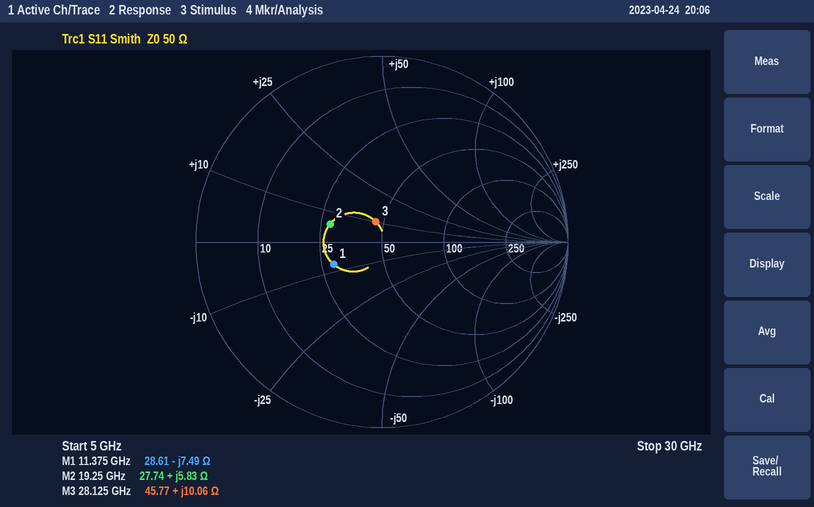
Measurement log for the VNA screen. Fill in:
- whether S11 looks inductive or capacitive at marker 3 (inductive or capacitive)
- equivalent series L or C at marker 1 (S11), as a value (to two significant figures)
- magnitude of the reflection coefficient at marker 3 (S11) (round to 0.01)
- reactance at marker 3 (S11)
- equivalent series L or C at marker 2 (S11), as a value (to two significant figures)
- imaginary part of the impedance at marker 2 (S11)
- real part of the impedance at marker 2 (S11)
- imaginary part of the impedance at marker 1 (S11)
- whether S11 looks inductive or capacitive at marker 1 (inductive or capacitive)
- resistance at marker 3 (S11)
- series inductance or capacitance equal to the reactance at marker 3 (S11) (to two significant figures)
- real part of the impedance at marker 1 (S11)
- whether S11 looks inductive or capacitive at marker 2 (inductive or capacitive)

inductive
1.9 pF
0.11
+10.06 Ω
48 pH
+5.83 Ω
27.74 Ω
-7.49 Ω
capacitive
45.77 Ω
57 pH
28.61 Ω
inductive
